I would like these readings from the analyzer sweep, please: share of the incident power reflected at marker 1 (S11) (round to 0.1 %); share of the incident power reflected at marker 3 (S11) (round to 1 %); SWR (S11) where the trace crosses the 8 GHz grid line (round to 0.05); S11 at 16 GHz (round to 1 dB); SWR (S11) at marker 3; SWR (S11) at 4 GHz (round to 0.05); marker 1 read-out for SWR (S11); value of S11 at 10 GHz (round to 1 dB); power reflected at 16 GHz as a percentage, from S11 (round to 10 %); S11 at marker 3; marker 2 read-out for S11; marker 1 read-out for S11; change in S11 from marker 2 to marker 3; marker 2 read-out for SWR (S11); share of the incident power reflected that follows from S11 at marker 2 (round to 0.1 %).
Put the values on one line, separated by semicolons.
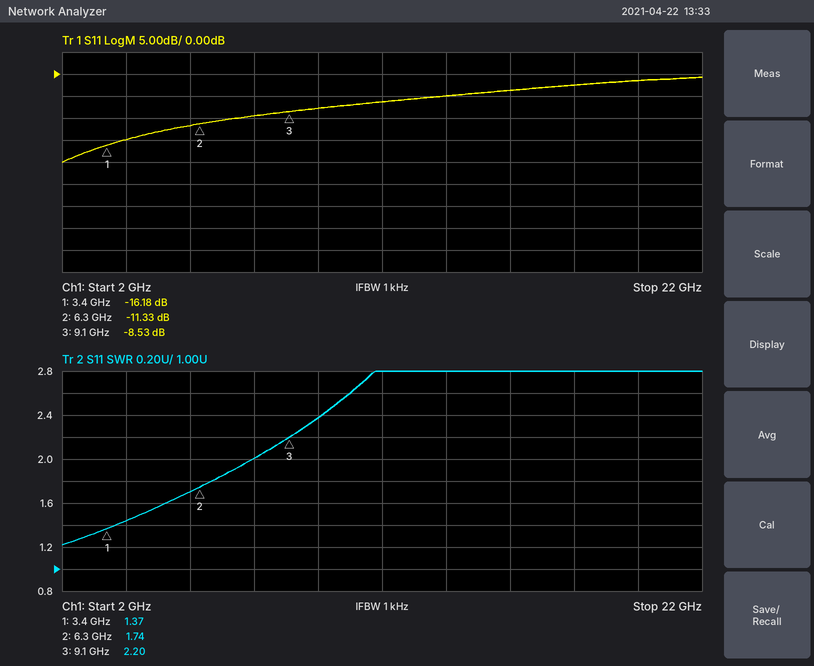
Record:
2.4 %; 14 %; 2.00; -4 dB; 2.20; 1.45; 1.37; -8 dB; 40 %; -8.53 dB; -11.33 dB; -16.18 dB; 2.80 dB; 1.74; 7.4 %
